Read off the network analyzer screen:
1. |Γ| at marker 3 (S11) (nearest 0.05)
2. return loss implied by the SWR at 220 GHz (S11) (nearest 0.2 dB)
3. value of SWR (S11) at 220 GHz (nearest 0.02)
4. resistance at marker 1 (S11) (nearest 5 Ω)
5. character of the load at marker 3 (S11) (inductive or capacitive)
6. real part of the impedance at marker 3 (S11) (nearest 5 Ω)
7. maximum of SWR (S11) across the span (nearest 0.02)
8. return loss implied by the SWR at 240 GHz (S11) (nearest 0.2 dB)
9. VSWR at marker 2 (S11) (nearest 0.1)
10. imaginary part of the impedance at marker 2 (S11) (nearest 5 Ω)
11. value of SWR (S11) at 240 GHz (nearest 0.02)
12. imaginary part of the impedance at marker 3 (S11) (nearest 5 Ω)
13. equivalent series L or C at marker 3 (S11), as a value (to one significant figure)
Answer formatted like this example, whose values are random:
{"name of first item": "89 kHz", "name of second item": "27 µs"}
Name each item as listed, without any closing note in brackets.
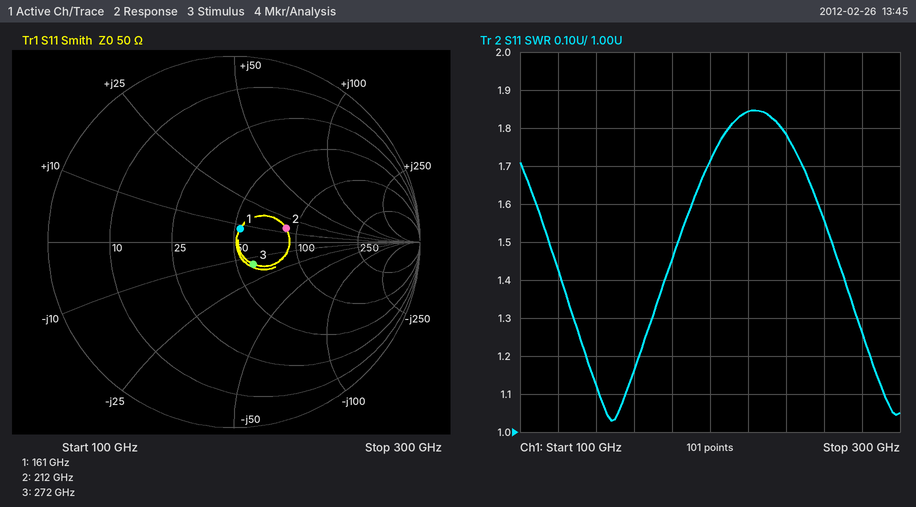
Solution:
{"|Γ| at marker 3 (S11)": "0.15", "return loss implied by the SWR at 220 GHz (S11)": "10.6 dB", "value of SWR (S11) at 220 GHz": "1.84", "resistance at marker 1 (S11)": "55 Ω", "character of the load at marker 3 (S11)": "capacitive", "real part of the impedance at marker 3 (S11)": "60 Ω", "maximum of SWR (S11) across the span": "1.84", "return loss implied by the SWR at 240 GHz (S11)": "11.0 dB", "VSWR at marker 2 (S11)": "1.8", "imaginary part of the impedance at marker 2 (S11)": "+15 Ω", "value of SWR (S11) at 240 GHz": "1.78", "imaginary part of the impedance at marker 3 (S11)": "-15 Ω", "equivalent series L or C at marker 3 (S11), as a value": "40 fF"}
